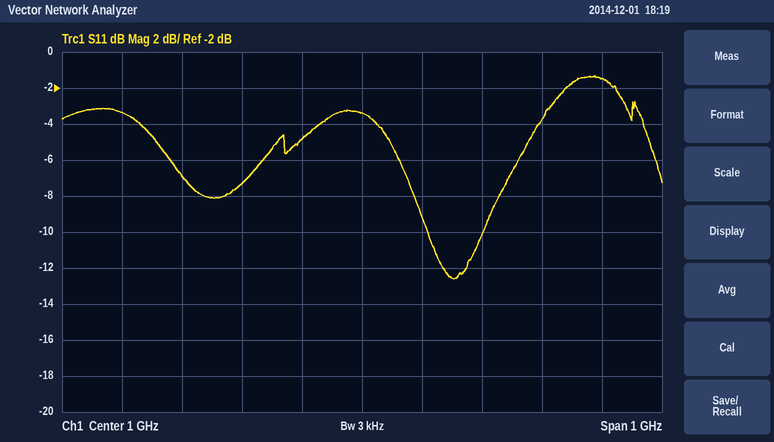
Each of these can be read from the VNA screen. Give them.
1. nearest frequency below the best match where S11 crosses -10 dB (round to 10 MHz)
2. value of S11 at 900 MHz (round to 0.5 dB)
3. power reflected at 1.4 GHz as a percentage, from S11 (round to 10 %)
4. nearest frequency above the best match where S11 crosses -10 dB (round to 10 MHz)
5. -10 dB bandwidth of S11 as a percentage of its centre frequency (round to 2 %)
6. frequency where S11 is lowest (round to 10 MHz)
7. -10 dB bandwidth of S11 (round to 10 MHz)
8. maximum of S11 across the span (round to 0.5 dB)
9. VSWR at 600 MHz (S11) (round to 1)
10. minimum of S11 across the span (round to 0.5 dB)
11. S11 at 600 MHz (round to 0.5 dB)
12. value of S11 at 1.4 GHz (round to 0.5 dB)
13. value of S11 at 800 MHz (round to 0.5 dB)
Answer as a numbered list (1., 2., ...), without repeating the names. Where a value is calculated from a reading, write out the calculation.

1. 1.11 GHz
2. -5.0 dB
3. 10^(-1.5/10) ≈ 70.8 %, so 70 % to the nearest 10 %
4. 1.20 GHz
5. 90 MHz / 1.155 GHz ≈ 8 %
6. 1.15 GHz
7. 1.20 GHz − 1.11 GHz = 90 MHz
8. -1.5 dB
9. |Γ| = 10^(-3.5/20) = 0.6683; VSWR = (1 + 0.6683)/(1 − 0.6683) ≈ 5
10. -12.5 dB
11. -3.5 dB
12. -1.5 dB
13. -7.5 dB
